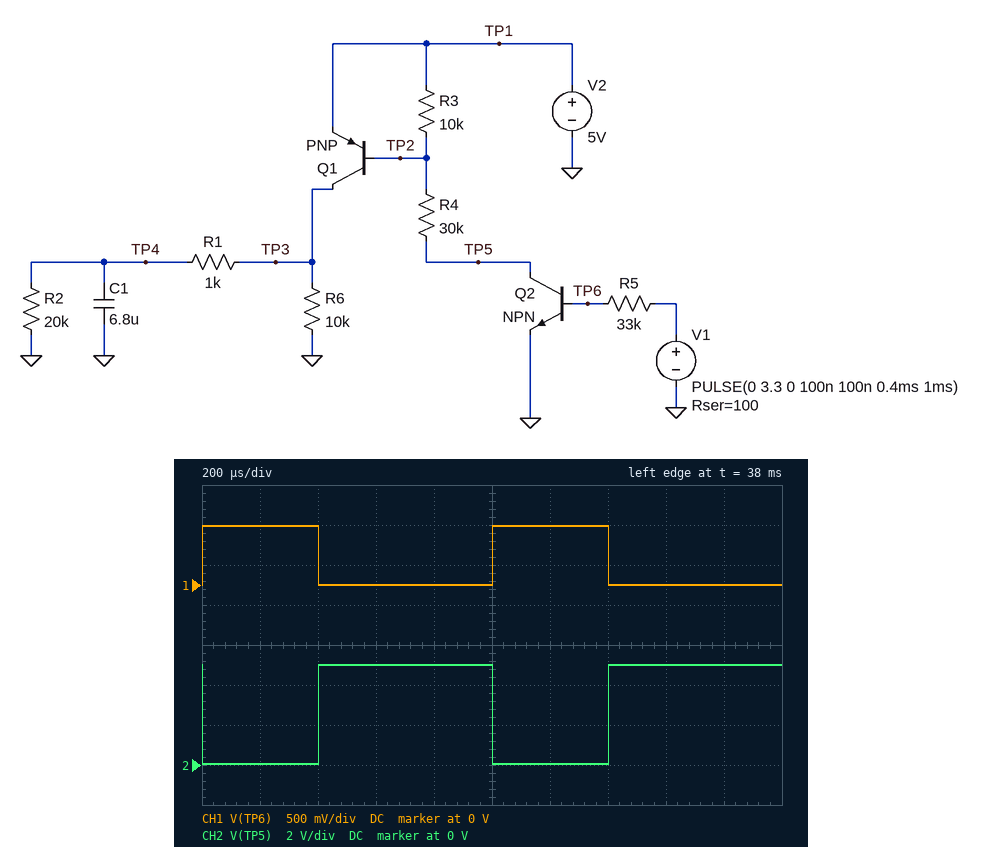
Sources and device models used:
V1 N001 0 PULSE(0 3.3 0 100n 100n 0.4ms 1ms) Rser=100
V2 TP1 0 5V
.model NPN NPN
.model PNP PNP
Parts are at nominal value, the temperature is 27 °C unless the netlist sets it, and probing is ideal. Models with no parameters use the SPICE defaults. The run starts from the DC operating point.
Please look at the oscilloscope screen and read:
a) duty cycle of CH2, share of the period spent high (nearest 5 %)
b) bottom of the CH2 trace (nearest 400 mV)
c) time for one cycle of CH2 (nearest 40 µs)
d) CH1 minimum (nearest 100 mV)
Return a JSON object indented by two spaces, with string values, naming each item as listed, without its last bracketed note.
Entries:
{
  "duty cycle of CH2, share of the period spent high": "60 %",
  "bottom of the CH2 trace": "0 V",
  "time for one cycle of CH2": "1.00 ms",
  "CH1 minimum": "0 V"
}
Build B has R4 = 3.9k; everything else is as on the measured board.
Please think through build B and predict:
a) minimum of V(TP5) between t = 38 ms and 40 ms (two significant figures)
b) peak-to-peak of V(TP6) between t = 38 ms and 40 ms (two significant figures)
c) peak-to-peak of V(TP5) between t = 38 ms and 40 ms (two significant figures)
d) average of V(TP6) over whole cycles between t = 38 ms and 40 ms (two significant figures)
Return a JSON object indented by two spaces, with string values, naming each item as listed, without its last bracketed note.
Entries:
{
  "minimum of V(TP5) between t = 38 ms and 40 ms": "75 mV",
  "peak-to-peak of V(TP6) between t = 38 ms and 40 ms": "780 mV",
  "peak-to-peak of V(TP5) between t = 38 ms and 40 ms": "4.9 V",
  "average of V(TP6) over whole cycles between t = 38 ms and 40 ms": "310 mV"
}
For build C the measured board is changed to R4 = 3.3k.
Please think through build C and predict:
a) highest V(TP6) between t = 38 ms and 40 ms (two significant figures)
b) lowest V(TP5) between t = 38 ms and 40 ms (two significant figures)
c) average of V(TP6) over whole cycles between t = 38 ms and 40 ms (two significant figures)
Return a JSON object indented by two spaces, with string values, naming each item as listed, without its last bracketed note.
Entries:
{
  "highest V(TP6) between t = 38 ms and 40 ms": "780 mV",
  "lowest V(TP5) between t = 38 ms and 40 ms": "80 mV",
  "average of V(TP6) over whole cycles between t = 38 ms and 40 ms": "310 mV"
}
